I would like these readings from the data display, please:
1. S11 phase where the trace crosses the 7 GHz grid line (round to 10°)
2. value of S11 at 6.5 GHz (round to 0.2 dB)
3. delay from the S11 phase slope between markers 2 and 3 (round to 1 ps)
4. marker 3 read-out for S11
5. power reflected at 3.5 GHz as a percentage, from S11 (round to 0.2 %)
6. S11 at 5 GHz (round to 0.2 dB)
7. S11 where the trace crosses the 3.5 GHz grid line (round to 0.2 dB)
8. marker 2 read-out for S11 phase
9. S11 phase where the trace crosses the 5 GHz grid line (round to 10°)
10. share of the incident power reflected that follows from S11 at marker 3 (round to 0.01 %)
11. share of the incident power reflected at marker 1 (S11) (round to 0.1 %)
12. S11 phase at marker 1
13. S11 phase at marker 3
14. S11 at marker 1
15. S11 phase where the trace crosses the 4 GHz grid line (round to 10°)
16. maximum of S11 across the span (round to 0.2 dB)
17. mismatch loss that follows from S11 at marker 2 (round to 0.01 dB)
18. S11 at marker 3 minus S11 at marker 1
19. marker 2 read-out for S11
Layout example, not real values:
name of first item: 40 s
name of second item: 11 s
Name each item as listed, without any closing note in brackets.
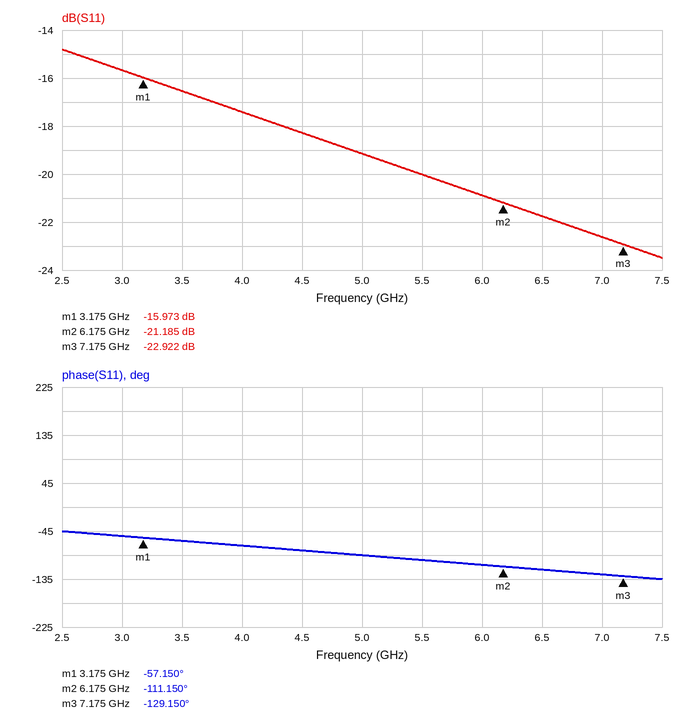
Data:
S11 phase where the trace crosses the 7 GHz grid line: -130°
value of S11 at 6.5 GHz: -21.8 dB
delay from the S11 phase slope between markers 2 and 3: 50 ps
marker 3 read-out for S11: -22.922 dB
power reflected at 3.5 GHz as a percentage, from S11: 2.2 %
S11 at 5 GHz: -19.2 dB
S11 where the trace crosses the 3.5 GHz grid line: -16.6 dB
marker 2 read-out for S11 phase: -111.150°
S11 phase where the trace crosses the 5 GHz grid line: -90°
share of the incident power reflected that follows from S11 at marker 3: 0.51 %
share of the incident power reflected at marker 1 (S11): 2.5 %
S11 phase at marker 1: -57.150°
S11 phase at marker 3: -129.150°
S11 at marker 1: -15.973 dB
S11 phase where the trace crosses the 4 GHz grid line: -70°
maximum of S11 across the span: -14.8 dB
mismatch loss that follows from S11 at marker 2: 0.03 dB
S11 at marker 3 minus S11 at marker 1: -6.949 dB
marker 2 read-out for S11: -21.185 dB
